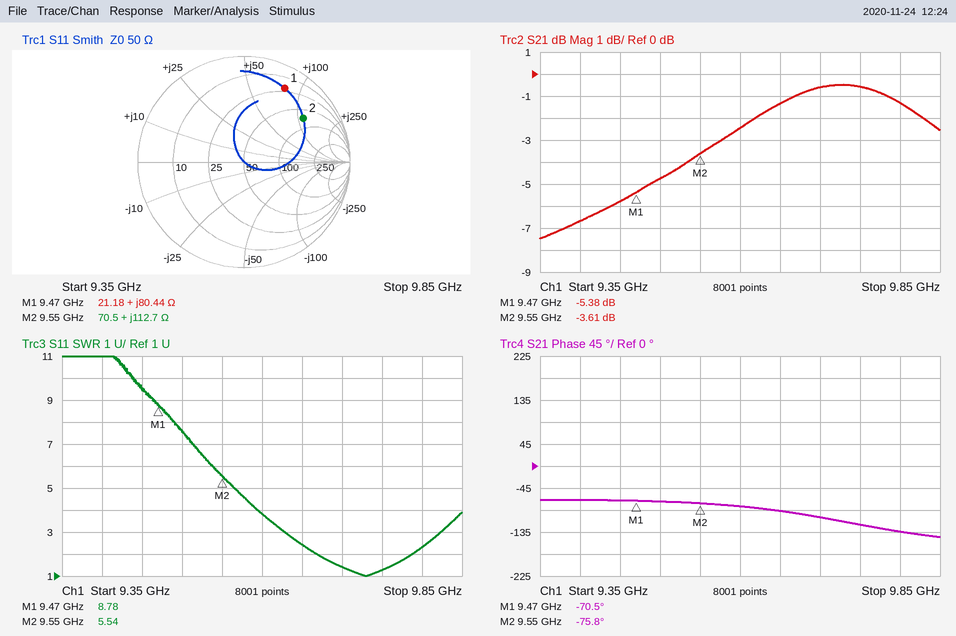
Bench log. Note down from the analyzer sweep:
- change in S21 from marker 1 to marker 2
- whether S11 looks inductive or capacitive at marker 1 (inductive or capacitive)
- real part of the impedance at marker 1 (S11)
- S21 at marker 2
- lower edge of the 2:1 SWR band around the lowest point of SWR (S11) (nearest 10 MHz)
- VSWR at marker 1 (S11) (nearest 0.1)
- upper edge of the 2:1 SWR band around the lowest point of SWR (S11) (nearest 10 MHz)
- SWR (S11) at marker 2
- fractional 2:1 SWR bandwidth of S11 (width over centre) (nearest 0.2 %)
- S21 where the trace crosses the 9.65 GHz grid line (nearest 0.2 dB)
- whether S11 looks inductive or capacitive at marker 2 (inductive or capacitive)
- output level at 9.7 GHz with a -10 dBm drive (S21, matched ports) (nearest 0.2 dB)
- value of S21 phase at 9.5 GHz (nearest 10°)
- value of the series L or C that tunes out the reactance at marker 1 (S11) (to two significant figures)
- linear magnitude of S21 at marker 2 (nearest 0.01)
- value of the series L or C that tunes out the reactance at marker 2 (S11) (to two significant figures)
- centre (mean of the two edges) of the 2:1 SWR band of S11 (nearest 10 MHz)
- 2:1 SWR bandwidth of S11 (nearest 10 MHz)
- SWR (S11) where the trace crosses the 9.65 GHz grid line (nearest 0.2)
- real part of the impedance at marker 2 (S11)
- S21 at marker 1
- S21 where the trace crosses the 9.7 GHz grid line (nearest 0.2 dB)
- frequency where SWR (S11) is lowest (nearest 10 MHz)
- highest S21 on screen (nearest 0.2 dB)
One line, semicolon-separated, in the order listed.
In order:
1.77 dB; inductive; 21.18 Ω; -3.61 dB; 9.67 GHz; 8.8; 9.79 GHz; 5.54; 1.2 %; -1.4 dB; inductive; -10.6 dBm; -70°; 210 fF; 0.66; 150 fF; 9.73 GHz; 120 MHz; 2.4; 70.5 Ω; -5.38 dB; -0.6 dB; 9.73 GHz; -0.4 dB
